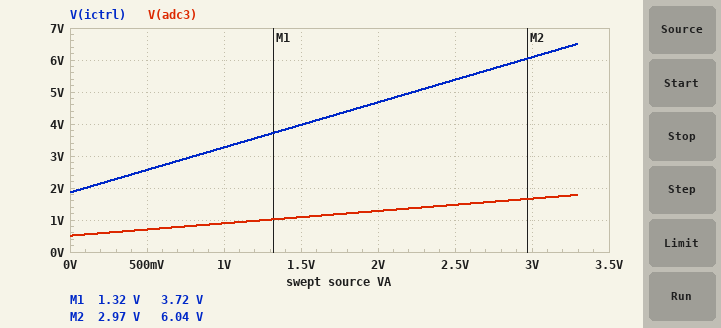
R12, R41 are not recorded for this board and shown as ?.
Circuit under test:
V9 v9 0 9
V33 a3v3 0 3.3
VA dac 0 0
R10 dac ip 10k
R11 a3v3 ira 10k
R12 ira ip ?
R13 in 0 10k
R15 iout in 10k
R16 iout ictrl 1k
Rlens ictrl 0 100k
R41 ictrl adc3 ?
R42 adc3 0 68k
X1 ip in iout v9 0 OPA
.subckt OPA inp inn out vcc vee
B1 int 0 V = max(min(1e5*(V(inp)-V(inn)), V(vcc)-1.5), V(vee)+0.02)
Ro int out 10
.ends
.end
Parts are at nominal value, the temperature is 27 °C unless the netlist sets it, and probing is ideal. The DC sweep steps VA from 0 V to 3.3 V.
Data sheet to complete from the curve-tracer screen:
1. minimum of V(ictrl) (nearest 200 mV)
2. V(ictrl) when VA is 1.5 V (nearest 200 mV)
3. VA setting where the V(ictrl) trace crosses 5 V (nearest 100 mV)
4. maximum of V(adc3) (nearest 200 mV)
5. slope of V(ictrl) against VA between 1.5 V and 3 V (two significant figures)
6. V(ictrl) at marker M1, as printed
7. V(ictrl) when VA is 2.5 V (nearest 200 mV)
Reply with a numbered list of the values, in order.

1. 1.8 V
2. 4.0 V
3. 2.2 V
4. 1.8 V
5. 1.4 V/V
6. 3.72 V
7. 5.4 V
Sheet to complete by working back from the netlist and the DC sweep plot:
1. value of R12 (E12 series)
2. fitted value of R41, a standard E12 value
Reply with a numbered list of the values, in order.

1. 15 kΩ
2. 180 kΩ
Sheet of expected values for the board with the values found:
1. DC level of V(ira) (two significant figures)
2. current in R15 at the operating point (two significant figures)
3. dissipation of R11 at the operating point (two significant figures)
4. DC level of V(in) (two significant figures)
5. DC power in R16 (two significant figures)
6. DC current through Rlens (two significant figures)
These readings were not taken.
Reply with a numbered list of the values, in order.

1. 2.4 V
2. 94 µA
3. 89 µW
4. 940 mV
5. 680 nW
6. 19 µA
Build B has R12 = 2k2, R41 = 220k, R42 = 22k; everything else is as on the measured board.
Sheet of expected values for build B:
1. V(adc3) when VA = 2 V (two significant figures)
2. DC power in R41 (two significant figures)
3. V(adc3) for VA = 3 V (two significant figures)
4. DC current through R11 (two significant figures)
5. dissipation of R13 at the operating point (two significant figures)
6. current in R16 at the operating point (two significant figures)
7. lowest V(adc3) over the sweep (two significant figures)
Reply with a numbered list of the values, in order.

1. 460 mV
2. 32 µW
3. 560 mV
4. 150 µA
5. 220 µW
6. 41 µA
7. 270 mV
